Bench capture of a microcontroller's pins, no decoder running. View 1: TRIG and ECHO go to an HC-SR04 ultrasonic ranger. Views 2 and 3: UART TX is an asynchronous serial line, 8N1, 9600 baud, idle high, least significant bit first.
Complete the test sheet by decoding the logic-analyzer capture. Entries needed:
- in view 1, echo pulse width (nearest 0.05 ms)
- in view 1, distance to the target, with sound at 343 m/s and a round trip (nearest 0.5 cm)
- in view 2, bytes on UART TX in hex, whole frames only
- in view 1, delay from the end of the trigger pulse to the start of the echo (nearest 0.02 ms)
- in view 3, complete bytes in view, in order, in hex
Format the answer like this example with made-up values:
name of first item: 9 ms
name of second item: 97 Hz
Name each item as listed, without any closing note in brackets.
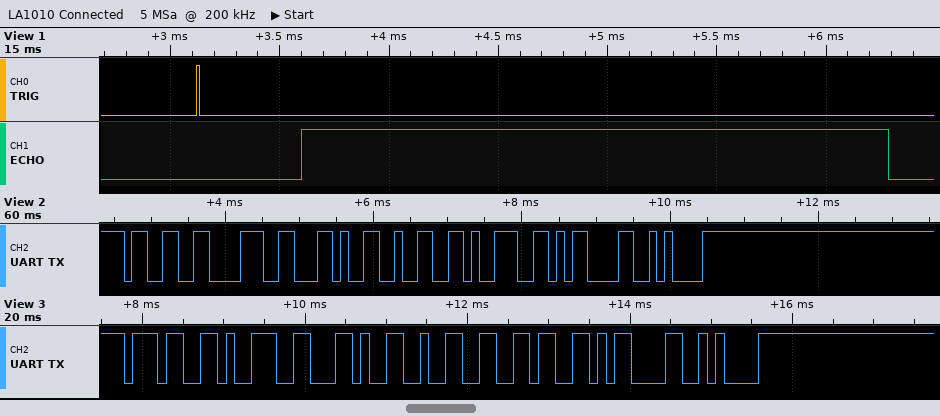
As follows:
in view 1, echo pulse width: 2.70 ms
in view 1, distance to the target, with sound at 343 m/s and a round trip: 46 cm
in view 2, bytes on UART TX in hex, whole frames only: 0x33 0x38 0x2C 0x32 0x39 0x0D 0x0A
in view 1, delay from the end of the trigger pulse to the start of the echo: 0.46 ms
in view 3, complete bytes in view, in order, in hex: 0x37 0x39 0x2C 0x32 0x36 0x0D 0x0A
